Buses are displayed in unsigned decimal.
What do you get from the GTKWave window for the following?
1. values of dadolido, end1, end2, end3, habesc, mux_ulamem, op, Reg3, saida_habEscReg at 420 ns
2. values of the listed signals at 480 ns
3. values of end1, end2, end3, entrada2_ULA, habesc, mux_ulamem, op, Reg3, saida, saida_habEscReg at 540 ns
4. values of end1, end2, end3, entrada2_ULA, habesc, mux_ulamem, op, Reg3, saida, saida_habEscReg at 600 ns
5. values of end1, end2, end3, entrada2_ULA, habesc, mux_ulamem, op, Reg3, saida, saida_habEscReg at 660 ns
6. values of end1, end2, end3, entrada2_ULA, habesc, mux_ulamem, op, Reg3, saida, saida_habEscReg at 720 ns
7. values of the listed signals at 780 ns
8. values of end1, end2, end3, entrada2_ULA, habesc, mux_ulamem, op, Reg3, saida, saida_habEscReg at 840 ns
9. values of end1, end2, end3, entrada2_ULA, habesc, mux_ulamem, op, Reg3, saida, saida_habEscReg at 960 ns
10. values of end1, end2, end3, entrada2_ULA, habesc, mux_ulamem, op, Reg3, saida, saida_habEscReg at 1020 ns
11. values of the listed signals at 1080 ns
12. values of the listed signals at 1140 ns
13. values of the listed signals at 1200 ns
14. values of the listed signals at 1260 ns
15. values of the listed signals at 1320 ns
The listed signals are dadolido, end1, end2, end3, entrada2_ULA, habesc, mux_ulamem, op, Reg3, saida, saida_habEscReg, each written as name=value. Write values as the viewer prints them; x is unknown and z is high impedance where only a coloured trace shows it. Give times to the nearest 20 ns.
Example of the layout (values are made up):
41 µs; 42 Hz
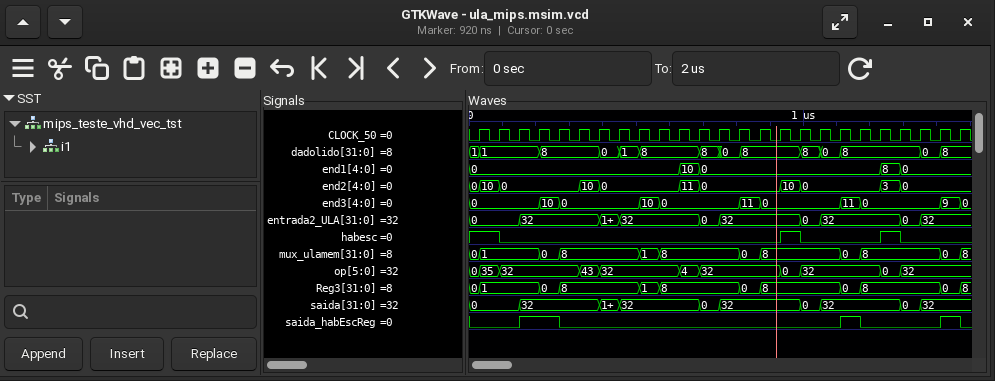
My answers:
dadolido=0, end1=0, end2=0, end3=0, habesc=0, mux_ulamem=8, op=32, Reg3=8, saida_habEscReg=0; dadolido=1, end1=0, end2=0, end3=0, entrada2_ULA=32, habesc=0, mux_ulamem=8, op=32, Reg3=8, saida=32, saida_habEscReg=0; end1=0, end2=0, end3=10, entrada2_ULA=32, habesc=0, mux_ulamem=1, op=32, Reg3=1, saida=32, saida_habEscReg=0; end1=0, end2=0, end3=0, entrada2_ULA=32, habesc=0, mux_ulamem=8, op=32, Reg3=8, saida=32, saida_habEscReg=0; end1=10, end2=11, end3=0, entrada2_ULA=32, habesc=0, mux_ulamem=8, op=4, Reg3=8, saida=32, saida_habEscReg=0; end1=0, end2=0, end3=0, entrada2_ULA=0, habesc=0, mux_ulamem=8, op=32, Reg3=8, saida=0, saida_habEscReg=0; dadolido=0, end1=0, end2=0, end3=0, entrada2_ULA=32, habesc=0, mux_ulamem=8, op=32, Reg3=8, saida=32, saida_habEscReg=0; end1=0, end2=0, end3=11, entrada2_ULA=32, habesc=0, mux_ulamem=0, op=32, Reg3=0, saida=32, saida_habEscReg=0; end1=0, end2=10, end3=0, entrada2_ULA=32, habesc=1, mux_ulamem=8, op=0, Reg3=8, saida=32, saida_habEscReg=0; end1=0, end2=0, end3=0, entrada2_ULA=0, habesc=0, mux_ulamem=8, op=32, Reg3=8, saida=0, saida_habEscReg=0; dadolido=0, end1=0, end2=0, end3=0, entrada2_ULA=32, habesc=0, mux_ulamem=8, op=32, Reg3=8, saida=32, saida_habEscReg=0; dadolido=8, end1=0, end2=0, end3=11, entrada2_ULA=32, habesc=0, mux_ulamem=0, op=32, Reg3=0, saida=32, saida_habEscReg=1; dadolido=8, end1=0, end2=0, end3=0, entrada2_ULA=32, habesc=0, mux_ulamem=8, op=32, Reg3=8, saida=32, saida_habEscReg=0; dadolido=8, end1=8, end2=3, end3=0, entrada2_ULA=32, habesc=1, mux_ulamem=8, op=0, Reg3=8, saida=32, saida_habEscReg=0; dadolido=8, end1=0, end2=0, end3=0, entrada2_ULA=0, habesc=0, mux_ulamem=8, op=32, Reg3=8, saida=0, saida_habEscReg=0
